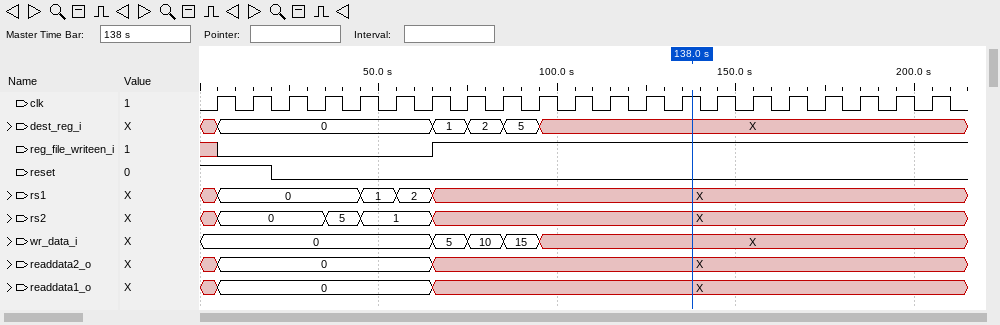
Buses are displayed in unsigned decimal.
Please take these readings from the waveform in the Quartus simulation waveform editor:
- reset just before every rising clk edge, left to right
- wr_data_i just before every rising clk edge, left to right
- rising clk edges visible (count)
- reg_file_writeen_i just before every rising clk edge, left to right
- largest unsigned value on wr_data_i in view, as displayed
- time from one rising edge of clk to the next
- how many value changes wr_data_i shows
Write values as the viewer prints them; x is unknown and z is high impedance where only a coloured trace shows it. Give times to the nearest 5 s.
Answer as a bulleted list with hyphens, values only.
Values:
- 1 1 0 0 0 0 0 0 0 0 0 0 0 0 0 0 0 0 0 0 0
- 0, 0, 0, 0, 0, 0, 0, 5, 10, 15, X, X, X, X, X, X, X, X, X, X, X
- 21
- x 0 0 0 0 0 0 1 1 1 1 1 1 1 1 1 1 1 1 1 1
- 15
- 10 s
- 4
